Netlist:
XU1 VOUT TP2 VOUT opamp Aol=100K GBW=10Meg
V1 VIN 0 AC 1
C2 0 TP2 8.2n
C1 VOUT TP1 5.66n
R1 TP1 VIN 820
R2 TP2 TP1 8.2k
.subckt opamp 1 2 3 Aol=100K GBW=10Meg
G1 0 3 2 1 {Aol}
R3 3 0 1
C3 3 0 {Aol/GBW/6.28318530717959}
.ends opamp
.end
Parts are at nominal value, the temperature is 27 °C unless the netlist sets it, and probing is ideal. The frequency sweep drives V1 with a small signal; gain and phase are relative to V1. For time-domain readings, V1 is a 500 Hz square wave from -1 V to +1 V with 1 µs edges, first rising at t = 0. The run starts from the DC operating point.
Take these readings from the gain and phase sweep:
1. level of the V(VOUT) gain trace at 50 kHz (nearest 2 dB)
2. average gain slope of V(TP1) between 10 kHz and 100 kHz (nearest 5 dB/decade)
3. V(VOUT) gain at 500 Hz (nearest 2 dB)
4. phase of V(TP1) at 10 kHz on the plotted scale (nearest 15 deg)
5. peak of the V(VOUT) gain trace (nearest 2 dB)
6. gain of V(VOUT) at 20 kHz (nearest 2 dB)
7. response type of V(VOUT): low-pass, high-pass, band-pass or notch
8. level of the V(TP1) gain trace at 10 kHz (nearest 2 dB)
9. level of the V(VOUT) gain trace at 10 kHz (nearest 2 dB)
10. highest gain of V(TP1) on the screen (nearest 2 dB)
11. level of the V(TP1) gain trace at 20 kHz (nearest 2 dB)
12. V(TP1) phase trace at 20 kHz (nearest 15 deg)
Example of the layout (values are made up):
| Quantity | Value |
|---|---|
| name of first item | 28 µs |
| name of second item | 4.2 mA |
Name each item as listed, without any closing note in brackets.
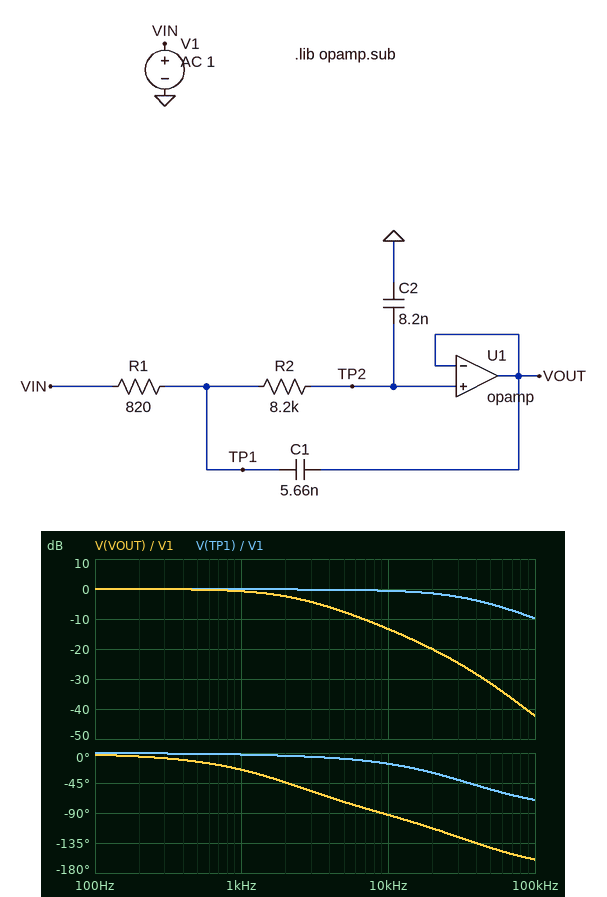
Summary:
| Quantity | Value |
|---|---|
| level of the V(VOUT) gain trace at 50 kHz | -32 dB |
| average gain slope of V(TP1) between 10 kHz and 100 kHz | -10 dB/decade |
| V(VOUT) gain at 500 Hz | 0 dB |
| phase of V(TP1) at 10 kHz on the plotted scale | -15 deg |
| peak of the V(VOUT) gain trace | 0 dB |
| gain of V(VOUT) at 20 kHz | -20 dB |
| response type of V(VOUT): low-pass, high-pass, band-pass or notch | low-pass |
| level of the V(TP1) gain trace at 10 kHz | 0 dB |
| level of the V(VOUT) gain trace at 10 kHz | -14 dB |
| highest gain of V(TP1) on the screen | 0 dB |
| level of the V(TP1) gain trace at 20 kHz | -2 dB |
| V(TP1) phase trace at 20 kHz | -30 deg |
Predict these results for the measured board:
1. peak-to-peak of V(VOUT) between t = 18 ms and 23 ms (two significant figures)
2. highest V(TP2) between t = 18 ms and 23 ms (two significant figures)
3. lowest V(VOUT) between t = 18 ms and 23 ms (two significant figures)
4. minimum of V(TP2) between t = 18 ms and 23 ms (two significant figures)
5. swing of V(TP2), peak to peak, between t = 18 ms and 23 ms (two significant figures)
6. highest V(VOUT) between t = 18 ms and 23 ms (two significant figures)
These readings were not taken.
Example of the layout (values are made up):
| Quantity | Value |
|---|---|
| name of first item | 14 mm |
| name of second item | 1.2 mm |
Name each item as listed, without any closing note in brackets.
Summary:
| Quantity | Value |
|---|---|
| peak-to-peak of V(VOUT) between t = 18 ms and 23 ms | 2.0 V |
| highest V(TP2) between t = 18 ms and 23 ms | 1.0 V |
| lowest V(VOUT) between t = 18 ms and 23 ms | -1.0 V |
| minimum of V(TP2) between t = 18 ms and 23 ms | -1.0 V |
| swing of V(TP2), peak to peak, between t = 18 ms and 23 ms | 2.0 V |
| highest V(VOUT) between t = 18 ms and 23 ms | 1.0 V |
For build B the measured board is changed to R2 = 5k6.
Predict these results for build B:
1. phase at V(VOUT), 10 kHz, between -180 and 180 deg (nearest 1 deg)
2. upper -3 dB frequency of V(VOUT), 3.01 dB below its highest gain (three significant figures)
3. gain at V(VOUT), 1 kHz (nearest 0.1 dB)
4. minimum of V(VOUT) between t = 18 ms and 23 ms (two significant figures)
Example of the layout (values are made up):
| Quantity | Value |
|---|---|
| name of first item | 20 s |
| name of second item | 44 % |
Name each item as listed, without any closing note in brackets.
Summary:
| Quantity | Value |
|---|---|
| phase at V(VOUT), 10 kHz, between -180 and 180 deg | -87 deg |
| upper -3 dB frequency of V(VOUT), 3.01 dB below its highest gain | 3.27 kHz |
| gain at V(VOUT), 1 kHz | -0.4 dB |
| minimum of V(VOUT) between t = 18 ms and 23 ms | -1.0 V |
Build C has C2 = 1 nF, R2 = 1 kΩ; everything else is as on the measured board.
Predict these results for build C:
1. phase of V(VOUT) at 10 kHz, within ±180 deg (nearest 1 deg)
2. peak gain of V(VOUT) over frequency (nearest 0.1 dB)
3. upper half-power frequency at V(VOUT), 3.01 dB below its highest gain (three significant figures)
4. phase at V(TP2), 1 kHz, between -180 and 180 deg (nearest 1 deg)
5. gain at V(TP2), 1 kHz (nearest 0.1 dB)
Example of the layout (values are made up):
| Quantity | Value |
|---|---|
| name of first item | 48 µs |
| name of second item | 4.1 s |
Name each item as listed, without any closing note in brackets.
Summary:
| Quantity | Value |
|---|---|
| phase of V(VOUT) at 10 kHz, within ±180 deg | -7 deg |
| peak gain of V(VOUT) over frequency | 2.4 dB |
| upper half-power frequency at V(VOUT), 3.01 dB below its highest gain | 87.0 kHz |
| phase at V(TP2), 1 kHz, between -180 and 180 deg | -1 deg |
| gain at V(TP2), 1 kHz | 0 dB |
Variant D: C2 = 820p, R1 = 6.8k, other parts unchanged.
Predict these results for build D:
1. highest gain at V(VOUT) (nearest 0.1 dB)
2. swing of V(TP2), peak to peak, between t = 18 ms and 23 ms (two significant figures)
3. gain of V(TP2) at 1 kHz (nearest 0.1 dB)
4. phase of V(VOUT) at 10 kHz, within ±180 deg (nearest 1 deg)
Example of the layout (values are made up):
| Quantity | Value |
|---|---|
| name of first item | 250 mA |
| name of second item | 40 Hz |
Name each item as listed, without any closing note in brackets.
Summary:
| Quantity | Value |
|---|---|
| highest gain at V(VOUT) | 3.0 dB |
| swing of V(TP2), peak to peak, between t = 18 ms and 23 ms | 3.1 V |
| gain of V(TP2) at 1 kHz | 0.1 dB |
| phase of V(VOUT) at 10 kHz, within ±180 deg | -92 deg |
